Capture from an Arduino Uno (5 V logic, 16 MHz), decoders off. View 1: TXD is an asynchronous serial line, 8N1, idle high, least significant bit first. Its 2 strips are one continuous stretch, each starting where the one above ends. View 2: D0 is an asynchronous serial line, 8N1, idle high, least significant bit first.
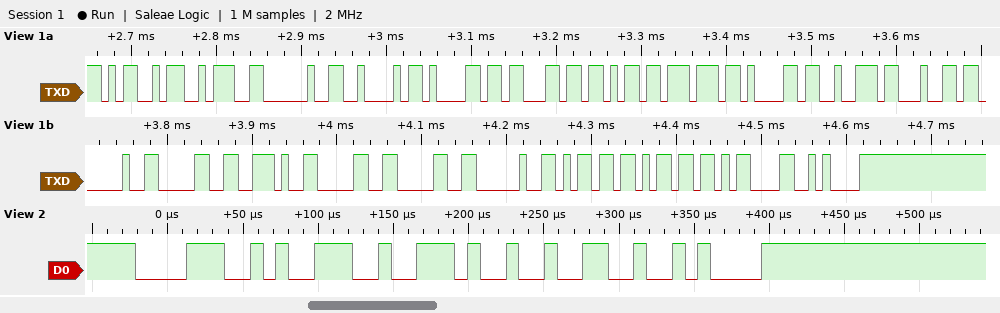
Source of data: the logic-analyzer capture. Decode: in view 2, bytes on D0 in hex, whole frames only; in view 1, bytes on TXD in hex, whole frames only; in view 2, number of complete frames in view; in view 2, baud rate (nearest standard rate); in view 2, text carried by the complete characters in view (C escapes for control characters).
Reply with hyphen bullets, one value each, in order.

- 38 39 2E 32 0A
- 0x4D 0x3A 0x20 0x42 0x61 0x63 0x6B 0x77 0x61 0x72 0x64 0x20 0x30 0x2E 0x30 0x30 0x20 0x6D 0x6D 0x0D 0x0A
- 5
- 115200 baud
- "89.2\n"
